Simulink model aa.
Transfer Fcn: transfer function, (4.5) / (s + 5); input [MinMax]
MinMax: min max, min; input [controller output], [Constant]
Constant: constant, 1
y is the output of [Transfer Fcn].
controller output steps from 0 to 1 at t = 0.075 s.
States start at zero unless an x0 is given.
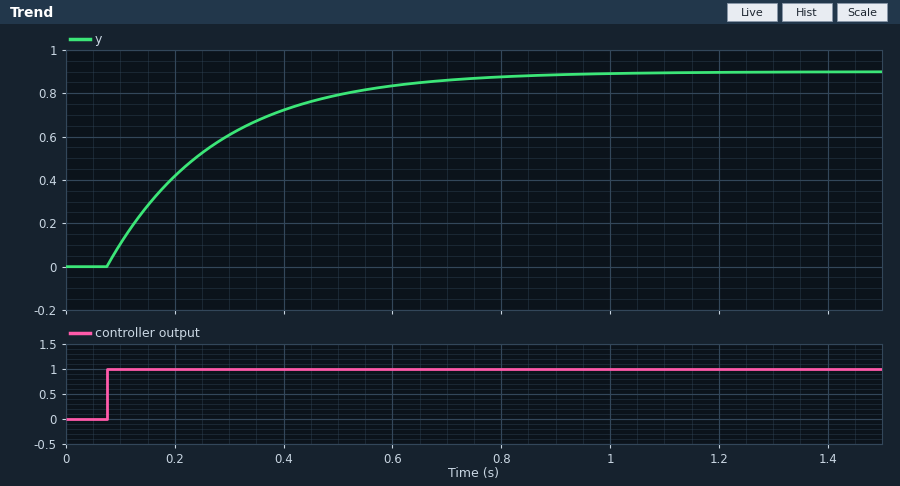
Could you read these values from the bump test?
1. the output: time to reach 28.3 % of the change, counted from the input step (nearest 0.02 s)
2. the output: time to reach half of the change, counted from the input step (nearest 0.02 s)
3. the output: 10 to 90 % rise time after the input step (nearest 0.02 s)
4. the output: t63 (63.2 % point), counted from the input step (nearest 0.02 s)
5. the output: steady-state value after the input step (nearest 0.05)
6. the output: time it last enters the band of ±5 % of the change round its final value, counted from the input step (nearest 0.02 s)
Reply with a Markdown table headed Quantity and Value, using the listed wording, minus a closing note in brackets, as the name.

| Quantity | Value |
|---|---|
| the output: time to reach 28.3 % of the change, counted from the input step | 0.06 s |
| the output: time to reach half of the change, counted from the input step | 0.14 s |
| the output: 10 to 90 % rise time after the input step | 0.44 s |
| the output: t63 (63.2 % point), counted from the input step | 0.20 s |
| the output: steady-state value after the input step | 0.90 |
| the output: time it last enters the band of ±5 % of the change round its final value, counted from the input step | 0.60 s |
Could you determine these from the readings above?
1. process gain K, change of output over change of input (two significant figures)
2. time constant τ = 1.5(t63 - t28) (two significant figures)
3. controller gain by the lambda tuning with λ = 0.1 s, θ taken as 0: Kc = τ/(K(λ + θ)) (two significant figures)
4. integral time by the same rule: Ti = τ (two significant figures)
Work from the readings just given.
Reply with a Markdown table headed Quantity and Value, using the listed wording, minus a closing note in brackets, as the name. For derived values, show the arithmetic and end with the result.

| Quantity | Value |
|---|---|
| process gain K, change of output over change of input | (0.9 - 0) / 1 = 0.90 |
| time constant τ = 1.5(t63 - t28) | 1.5 × (0.2 - 0.06) = 0.21 s |
| controller gain by the lambda tuning with λ = 0.1 s, θ taken as 0: Kc = τ/(K(λ + θ)) | 0.21 / (0.9 × (0.1 + 0)) = 2.3 |
| integral time by the same rule: Ti = τ | 0.21 s |
